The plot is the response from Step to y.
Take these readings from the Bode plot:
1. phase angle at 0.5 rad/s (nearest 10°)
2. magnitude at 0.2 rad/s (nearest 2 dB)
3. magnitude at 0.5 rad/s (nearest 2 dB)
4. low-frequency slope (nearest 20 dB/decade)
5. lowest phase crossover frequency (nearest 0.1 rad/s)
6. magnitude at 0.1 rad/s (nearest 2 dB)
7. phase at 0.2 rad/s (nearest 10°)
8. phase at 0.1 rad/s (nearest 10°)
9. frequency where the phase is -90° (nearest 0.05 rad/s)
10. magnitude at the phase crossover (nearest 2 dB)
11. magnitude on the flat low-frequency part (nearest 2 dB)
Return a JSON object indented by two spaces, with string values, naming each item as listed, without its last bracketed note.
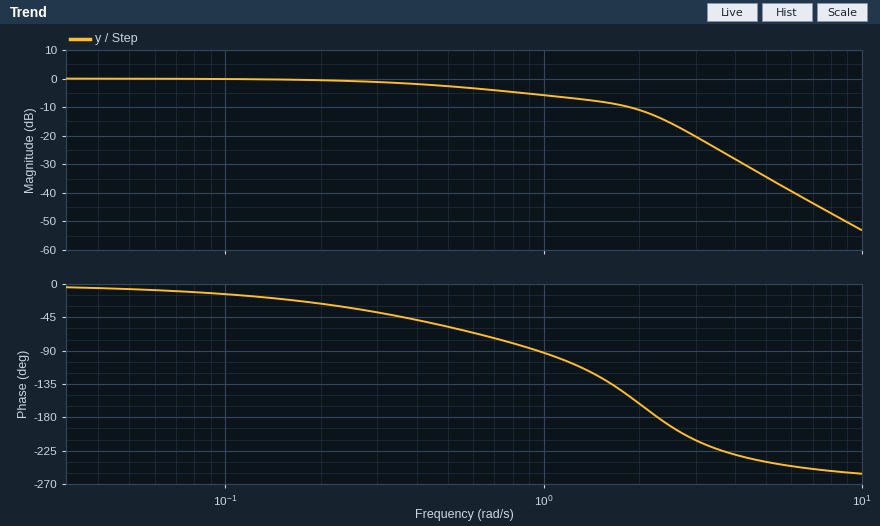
{
  "phase angle at 0.5 rad/s": "-60°",
  "magnitude at 0.2 rad/s": "0 dB",
  "magnitude at 0.5 rad/s": "-2 dB",
  "low-frequency slope": "0 dB/decade",
  "lowest phase crossover frequency": "2.3 rad/s",
  "magnitude at 0.1 rad/s": "0 dB",
  "phase at 0.2 rad/s": "-30°",
  "phase at 0.1 rad/s": "-10°",
  "frequency where the phase is -90°": "0.95 rad/s",
  "magnitude at the phase crossover": "-14 dB",
  "magnitude on the flat low-frequency part": "0 dB"
}
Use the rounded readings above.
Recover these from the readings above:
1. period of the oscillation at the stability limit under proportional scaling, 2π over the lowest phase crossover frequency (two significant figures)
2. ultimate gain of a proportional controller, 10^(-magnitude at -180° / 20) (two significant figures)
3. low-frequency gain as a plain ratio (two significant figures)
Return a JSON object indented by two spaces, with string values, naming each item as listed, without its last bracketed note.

{
  "period of the oscillation at the stability limit under proportional scaling, 2π over the lowest phase crossover frequency": "2.7 s",
  "ultimate gain of a proportional controller, 10^(-magnitude at -180° / 20)": "5.0",
  "low-frequency gain as a plain ratio": "1.0"
}
